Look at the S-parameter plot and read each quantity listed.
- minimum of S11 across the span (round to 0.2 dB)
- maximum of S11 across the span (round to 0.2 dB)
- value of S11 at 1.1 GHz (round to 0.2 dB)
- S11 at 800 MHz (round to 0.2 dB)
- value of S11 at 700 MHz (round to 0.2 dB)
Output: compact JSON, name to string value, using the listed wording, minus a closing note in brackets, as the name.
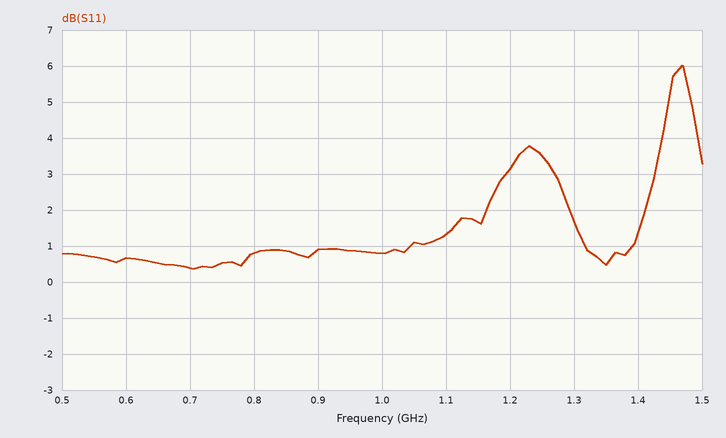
{"minimum of S11 across the span": "0.4 dB", "maximum of S11 across the span": "6.0 dB", "value of S11 at 1.1 GHz": "1.4 dB", "S11 at 800 MHz": "0.8 dB", "value of S11 at 700 MHz": "0.4 dB"}
